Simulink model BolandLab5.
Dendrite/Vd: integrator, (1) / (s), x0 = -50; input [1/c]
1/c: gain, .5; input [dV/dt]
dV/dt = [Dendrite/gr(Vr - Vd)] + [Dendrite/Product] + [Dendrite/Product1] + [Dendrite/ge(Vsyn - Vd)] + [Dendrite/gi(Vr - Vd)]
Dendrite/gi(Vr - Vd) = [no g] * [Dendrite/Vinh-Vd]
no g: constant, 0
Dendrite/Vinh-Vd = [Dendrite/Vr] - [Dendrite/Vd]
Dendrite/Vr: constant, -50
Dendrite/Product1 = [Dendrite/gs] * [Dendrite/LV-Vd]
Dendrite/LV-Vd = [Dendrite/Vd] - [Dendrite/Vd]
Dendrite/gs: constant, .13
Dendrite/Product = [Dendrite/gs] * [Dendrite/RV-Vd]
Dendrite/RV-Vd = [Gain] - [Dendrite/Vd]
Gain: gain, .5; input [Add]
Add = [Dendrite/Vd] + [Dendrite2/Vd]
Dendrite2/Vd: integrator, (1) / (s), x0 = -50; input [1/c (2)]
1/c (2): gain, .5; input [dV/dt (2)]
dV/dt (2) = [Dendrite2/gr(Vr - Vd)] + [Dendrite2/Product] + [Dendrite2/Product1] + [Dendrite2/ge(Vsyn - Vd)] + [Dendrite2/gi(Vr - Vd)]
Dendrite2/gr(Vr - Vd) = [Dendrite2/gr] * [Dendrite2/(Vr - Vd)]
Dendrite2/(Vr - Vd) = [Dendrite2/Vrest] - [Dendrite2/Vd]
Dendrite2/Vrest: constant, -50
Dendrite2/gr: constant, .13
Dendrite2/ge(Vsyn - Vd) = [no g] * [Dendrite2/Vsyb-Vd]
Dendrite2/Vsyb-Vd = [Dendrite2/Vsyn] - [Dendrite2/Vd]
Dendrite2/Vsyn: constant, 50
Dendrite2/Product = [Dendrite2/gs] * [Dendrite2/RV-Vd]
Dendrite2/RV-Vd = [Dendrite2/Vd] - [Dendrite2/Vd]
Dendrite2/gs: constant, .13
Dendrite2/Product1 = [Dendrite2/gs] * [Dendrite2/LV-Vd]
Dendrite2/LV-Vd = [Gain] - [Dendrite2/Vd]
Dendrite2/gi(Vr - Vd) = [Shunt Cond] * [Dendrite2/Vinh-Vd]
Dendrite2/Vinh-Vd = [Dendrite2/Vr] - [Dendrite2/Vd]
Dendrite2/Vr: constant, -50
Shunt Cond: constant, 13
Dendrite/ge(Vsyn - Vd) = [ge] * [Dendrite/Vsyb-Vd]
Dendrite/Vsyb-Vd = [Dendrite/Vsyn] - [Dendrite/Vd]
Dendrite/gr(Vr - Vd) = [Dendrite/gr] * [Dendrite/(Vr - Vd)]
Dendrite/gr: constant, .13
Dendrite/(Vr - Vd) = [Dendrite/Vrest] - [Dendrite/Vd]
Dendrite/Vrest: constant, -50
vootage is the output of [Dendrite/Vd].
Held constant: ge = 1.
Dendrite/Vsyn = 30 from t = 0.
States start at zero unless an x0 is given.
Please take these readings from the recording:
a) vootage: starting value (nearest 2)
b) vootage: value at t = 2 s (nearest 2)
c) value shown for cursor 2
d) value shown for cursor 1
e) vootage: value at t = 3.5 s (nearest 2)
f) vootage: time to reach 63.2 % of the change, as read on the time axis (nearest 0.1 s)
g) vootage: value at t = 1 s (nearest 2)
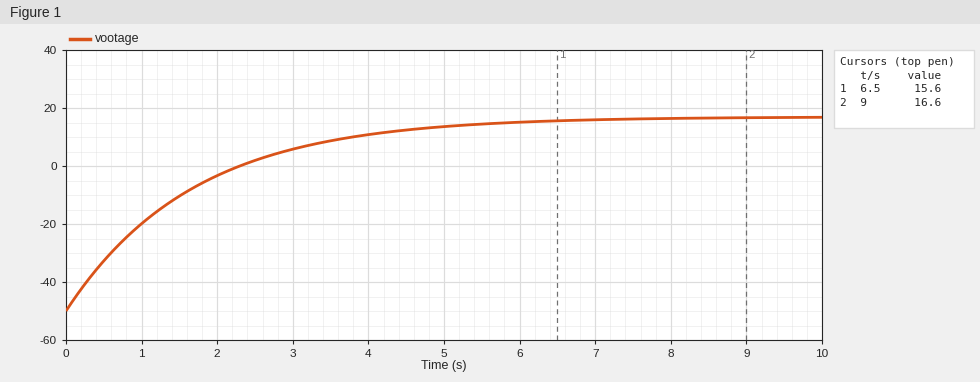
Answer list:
-50
-4
16.6
15.6
8
1.7 s
-20
